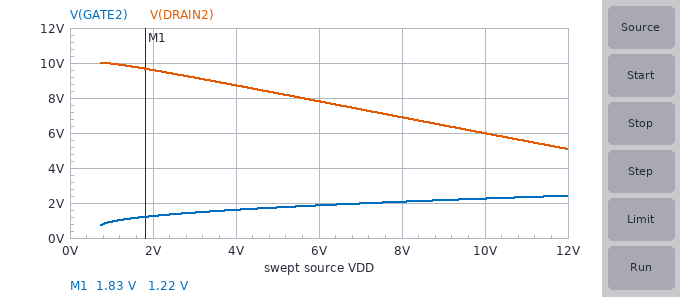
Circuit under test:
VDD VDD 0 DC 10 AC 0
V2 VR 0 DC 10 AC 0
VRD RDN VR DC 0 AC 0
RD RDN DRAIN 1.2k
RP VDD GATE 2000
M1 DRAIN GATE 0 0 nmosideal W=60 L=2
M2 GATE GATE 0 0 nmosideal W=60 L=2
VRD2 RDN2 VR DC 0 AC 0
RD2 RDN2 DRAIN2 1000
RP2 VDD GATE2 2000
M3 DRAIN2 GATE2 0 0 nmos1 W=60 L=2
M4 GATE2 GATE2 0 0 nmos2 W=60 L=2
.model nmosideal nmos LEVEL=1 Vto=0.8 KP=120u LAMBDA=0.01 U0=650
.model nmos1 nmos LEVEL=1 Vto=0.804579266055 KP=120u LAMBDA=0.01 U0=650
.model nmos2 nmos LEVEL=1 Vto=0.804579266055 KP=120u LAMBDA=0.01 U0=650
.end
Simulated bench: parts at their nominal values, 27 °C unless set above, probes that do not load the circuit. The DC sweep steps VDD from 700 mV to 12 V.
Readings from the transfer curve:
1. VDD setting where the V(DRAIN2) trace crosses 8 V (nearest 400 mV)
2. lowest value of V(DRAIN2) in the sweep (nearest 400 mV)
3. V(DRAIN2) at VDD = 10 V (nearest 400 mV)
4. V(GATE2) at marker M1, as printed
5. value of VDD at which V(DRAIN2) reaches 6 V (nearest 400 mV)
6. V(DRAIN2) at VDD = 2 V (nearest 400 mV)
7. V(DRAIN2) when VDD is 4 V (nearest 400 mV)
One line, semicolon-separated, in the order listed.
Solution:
5.6 V; 5.2 V; 6.0 V; 1.22 V; 10.0 V; 9.6 V; 8.8 V
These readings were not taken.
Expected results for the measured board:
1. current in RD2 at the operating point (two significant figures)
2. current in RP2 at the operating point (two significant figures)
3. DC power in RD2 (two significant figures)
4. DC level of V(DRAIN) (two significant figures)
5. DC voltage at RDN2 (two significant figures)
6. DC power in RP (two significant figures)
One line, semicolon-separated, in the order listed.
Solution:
4.0 mA; 3.9 mA; 16 mW; 5.2 V; 10 V; 30 mW
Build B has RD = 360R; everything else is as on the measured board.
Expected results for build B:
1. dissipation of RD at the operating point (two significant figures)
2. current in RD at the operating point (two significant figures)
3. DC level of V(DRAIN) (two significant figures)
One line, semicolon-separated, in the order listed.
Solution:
6.1 mW; 4.1 mA; 8.5 V
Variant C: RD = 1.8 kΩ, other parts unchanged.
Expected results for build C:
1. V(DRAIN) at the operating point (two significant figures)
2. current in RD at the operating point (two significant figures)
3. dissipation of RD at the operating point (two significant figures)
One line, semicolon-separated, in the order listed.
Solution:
3.0 V; 3.9 mA; 27 mW
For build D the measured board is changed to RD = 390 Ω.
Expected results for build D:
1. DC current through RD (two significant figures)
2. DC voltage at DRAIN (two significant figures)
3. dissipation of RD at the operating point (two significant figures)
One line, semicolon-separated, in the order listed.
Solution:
4.1 mA; 8.4 V; 6.6 mW
